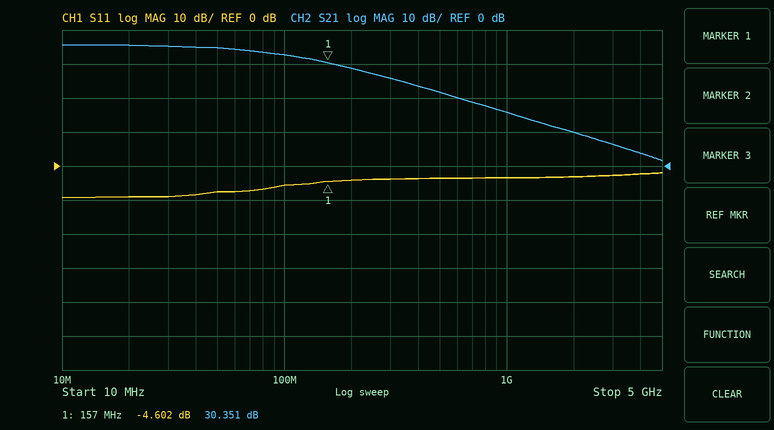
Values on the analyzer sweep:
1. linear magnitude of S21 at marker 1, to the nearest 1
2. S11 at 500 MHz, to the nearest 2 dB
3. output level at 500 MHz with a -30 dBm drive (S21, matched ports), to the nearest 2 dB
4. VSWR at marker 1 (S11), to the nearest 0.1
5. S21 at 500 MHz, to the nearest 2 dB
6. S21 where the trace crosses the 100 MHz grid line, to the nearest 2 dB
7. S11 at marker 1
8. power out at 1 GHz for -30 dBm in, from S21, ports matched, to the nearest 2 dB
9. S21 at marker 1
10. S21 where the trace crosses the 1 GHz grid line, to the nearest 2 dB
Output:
33
-4 dB
-8 dBm
3.9
22 dB
32 dB
-4.602 dB
-14 dBm
30.351 dB
16 dB
